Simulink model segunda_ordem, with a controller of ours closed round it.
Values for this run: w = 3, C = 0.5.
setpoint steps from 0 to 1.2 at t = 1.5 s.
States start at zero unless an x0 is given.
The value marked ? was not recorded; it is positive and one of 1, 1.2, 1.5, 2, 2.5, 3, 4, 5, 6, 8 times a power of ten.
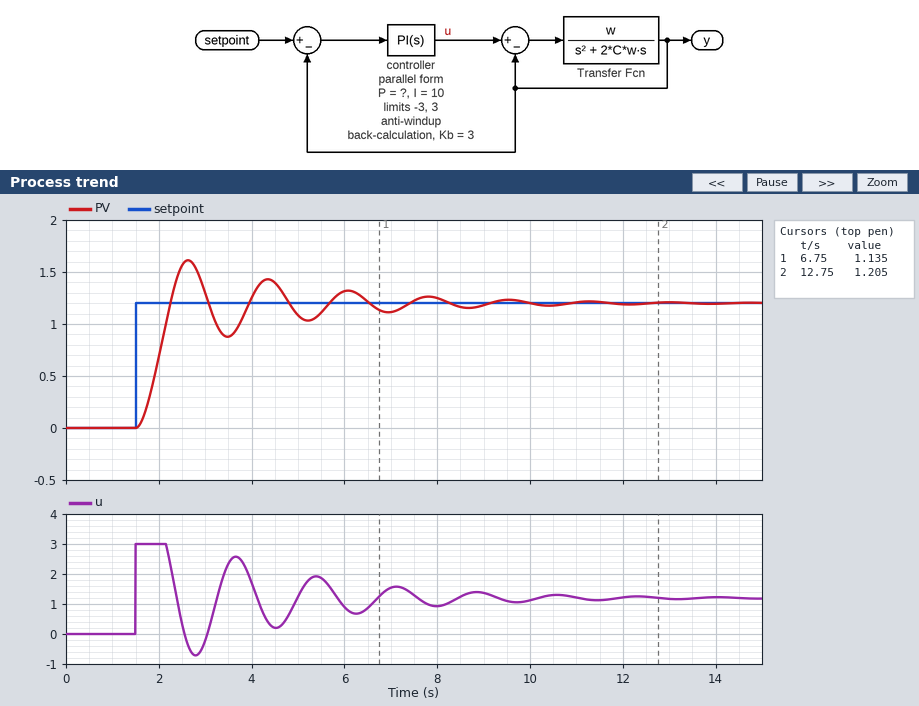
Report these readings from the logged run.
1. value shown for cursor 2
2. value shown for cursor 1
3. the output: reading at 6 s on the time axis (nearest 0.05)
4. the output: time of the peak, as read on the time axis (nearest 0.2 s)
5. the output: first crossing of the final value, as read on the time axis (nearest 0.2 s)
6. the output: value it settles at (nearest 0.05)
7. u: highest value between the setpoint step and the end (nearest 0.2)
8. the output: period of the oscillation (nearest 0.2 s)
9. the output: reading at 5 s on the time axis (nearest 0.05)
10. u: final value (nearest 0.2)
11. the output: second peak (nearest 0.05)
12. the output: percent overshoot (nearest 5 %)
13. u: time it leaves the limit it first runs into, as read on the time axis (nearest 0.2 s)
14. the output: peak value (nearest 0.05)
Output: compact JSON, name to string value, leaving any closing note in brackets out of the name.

{"value shown for cursor 2": "1.205", "value shown for cursor 1": "1.135", "the output: reading at 6 s on the time axis": "1.30", "the output: time of the peak, as read on the time axis": "2.6 s", "the output: first crossing of the final value, as read on the time axis": "2.2 s", "the output: value it settles at": "1.20", "u: highest value between the setpoint step and the end": "3.0", "the output: period of the oscillation": "1.8 s", "the output: reading at 5 s on the time axis": "1.10", "u: final value": "1.2", "the output: second peak": "1.45", "the output: percent overshoot": "35 %", "u: time it leaves the limit it first runs into, as read on the time axis": "2.2 s", "the output: peak value": "1.60"}
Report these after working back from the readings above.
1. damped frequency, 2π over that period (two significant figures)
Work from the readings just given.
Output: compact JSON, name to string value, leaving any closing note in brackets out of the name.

{"damped frequency, 2π over that period": "3.5 rad/s"}
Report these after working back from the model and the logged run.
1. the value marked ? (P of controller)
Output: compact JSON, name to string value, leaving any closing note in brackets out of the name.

{"the value marked ?": "4"}
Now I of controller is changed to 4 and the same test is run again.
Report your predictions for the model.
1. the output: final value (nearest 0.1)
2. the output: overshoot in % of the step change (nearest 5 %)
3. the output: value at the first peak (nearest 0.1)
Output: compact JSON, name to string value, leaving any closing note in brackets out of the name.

{"the output: final value": "1.2", "the output: overshoot in % of the step change": "10 %", "the output: value at the first peak": "1.3"}
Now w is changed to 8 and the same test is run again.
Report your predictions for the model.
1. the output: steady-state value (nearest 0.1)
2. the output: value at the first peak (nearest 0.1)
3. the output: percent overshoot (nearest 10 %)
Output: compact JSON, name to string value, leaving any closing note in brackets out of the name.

{"the output: steady-state value": "1.2", "the output: value at the first peak": "1.4", "the output: percent overshoot": "20 %"}
